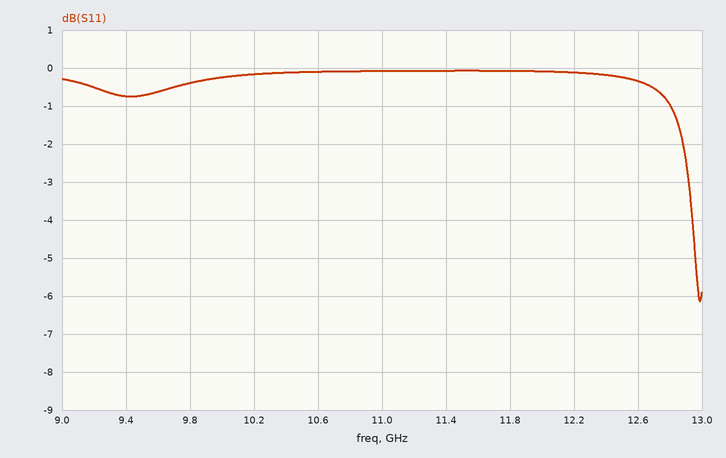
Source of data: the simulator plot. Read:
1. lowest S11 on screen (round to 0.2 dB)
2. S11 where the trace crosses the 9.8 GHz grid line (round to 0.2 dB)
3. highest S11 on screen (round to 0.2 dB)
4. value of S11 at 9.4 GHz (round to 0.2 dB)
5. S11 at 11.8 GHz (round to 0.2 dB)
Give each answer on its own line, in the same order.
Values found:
-6.2 dB
-0.4 dB
0.0 dB
-0.8 dB
0.0 dB
